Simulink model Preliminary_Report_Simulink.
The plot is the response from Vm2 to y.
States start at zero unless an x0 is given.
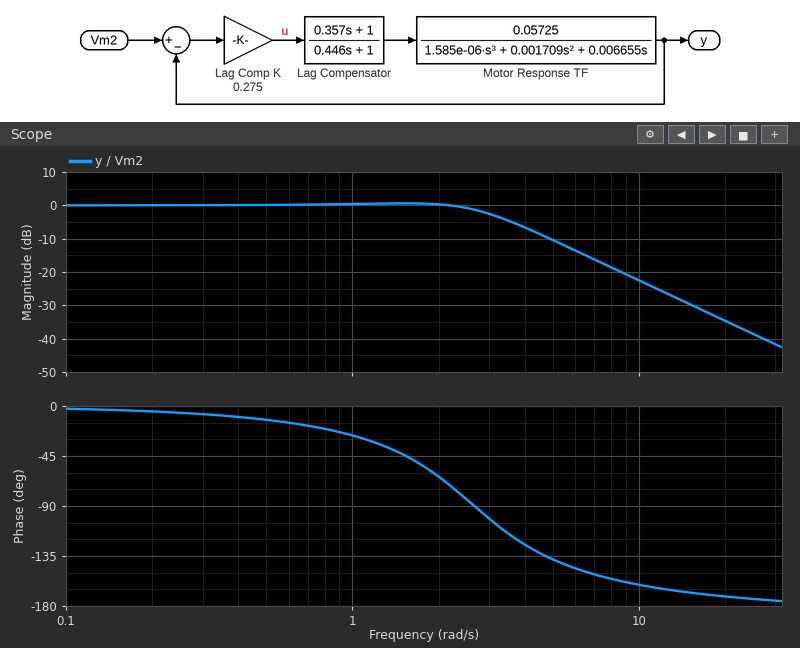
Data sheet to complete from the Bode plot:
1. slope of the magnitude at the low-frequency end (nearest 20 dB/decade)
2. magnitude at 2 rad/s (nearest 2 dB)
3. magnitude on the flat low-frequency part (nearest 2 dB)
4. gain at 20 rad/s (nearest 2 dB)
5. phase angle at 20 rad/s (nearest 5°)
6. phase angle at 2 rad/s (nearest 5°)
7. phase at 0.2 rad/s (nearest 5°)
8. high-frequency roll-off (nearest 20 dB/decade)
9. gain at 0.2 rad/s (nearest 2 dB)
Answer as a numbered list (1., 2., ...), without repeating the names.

1. 0 dB/decade
2. 0 dB
3. 0 dB
4. -34 dB
5. -170°
6. -65°
7. -5°
8. -40 dB/decade
9. 0 dB
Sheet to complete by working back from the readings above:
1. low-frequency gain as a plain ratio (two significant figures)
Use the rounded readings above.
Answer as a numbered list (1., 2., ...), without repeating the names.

1. 1.0
